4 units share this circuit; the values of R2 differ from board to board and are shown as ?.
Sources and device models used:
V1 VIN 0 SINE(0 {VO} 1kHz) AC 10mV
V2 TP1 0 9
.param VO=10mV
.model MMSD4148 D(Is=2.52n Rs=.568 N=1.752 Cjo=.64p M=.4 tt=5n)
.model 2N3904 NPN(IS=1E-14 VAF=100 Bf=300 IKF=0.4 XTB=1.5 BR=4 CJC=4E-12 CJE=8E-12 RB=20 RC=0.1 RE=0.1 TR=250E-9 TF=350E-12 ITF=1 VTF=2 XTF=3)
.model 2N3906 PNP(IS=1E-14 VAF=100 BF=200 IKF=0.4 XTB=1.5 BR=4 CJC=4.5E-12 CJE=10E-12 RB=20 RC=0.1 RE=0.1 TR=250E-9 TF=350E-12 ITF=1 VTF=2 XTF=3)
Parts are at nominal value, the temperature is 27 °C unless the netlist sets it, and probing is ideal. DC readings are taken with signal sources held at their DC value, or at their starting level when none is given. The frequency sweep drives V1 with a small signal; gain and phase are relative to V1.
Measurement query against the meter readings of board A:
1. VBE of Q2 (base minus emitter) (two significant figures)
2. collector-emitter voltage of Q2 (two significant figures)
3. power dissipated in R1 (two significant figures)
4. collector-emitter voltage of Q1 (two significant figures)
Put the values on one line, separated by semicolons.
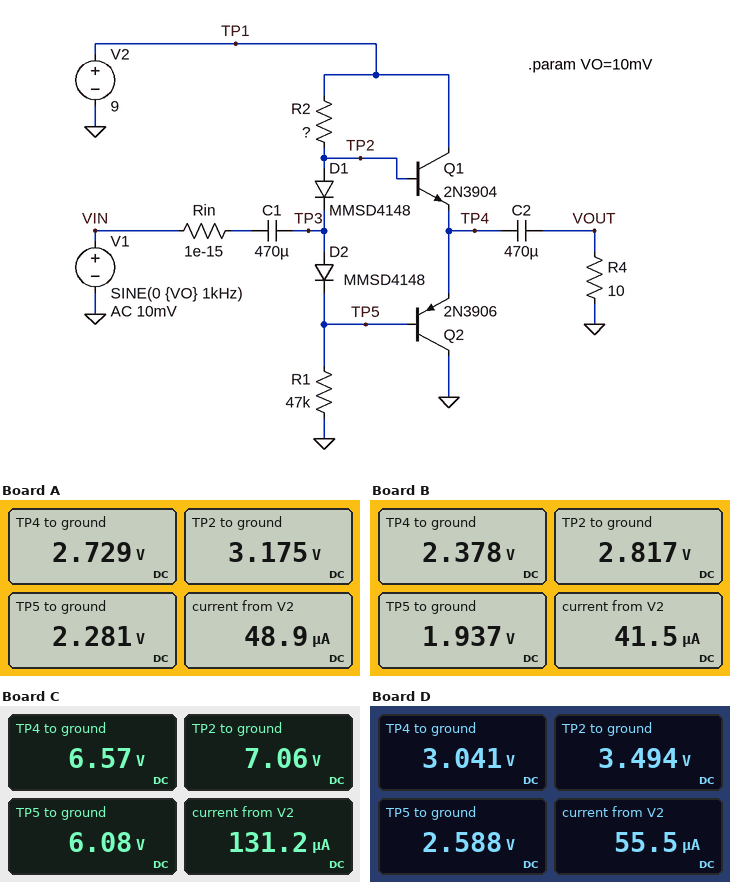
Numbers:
-450 mV; -2.7 V; 110 µW; 6.3 V
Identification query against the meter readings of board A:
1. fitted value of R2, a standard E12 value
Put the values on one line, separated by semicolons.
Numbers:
120 kΩ
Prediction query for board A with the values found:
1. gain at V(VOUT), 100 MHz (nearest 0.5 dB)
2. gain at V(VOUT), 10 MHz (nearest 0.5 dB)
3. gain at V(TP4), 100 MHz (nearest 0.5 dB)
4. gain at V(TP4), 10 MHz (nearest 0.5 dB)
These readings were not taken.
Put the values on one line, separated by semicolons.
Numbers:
-27.0 dB; -40.0 dB; -27.0 dB; -40.0 dB
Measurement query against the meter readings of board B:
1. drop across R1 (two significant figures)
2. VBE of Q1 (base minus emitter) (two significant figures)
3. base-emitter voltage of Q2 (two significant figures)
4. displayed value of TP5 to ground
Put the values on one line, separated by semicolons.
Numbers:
1.9 V; 440 mV; -440 mV; 1.937 V
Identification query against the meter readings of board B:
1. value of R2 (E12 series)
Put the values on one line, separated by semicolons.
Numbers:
150 kΩ
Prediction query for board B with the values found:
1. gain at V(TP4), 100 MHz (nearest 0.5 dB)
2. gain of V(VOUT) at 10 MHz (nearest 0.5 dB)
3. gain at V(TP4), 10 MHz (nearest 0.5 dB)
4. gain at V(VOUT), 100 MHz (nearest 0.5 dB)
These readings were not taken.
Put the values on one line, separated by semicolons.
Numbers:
-27.5 dB; -40.5 dB; -40.5 dB; -27.5 dB
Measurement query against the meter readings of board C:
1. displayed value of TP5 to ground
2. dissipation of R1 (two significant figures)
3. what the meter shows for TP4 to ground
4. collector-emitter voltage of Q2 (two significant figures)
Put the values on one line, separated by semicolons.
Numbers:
6.08 V; 790 µW; 6.57 V; -6.6 V
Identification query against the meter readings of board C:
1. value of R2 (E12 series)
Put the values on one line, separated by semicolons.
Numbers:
15 kΩ
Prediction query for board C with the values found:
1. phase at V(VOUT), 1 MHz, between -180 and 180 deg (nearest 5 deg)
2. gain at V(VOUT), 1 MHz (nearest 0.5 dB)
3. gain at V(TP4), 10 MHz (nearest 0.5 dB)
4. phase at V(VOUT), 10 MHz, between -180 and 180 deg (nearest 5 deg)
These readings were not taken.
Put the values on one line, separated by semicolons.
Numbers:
45 deg; -53.5 dB; -37.5 dB; 70 deg
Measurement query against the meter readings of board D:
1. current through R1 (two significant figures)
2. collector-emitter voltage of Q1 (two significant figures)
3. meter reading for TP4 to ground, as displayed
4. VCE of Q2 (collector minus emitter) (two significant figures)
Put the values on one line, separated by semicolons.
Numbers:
55 µA; 6.0 V; 3.041 V; -3.0 V
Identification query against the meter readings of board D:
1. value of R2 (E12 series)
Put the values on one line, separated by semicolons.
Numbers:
100 kΩ
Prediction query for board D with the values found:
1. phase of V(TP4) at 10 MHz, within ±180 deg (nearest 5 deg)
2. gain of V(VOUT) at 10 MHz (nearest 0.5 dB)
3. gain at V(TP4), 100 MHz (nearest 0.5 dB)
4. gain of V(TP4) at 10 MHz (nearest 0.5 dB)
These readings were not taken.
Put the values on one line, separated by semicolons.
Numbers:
60 deg; -39.5 dB; -26.0 dB; -39.5 dB
